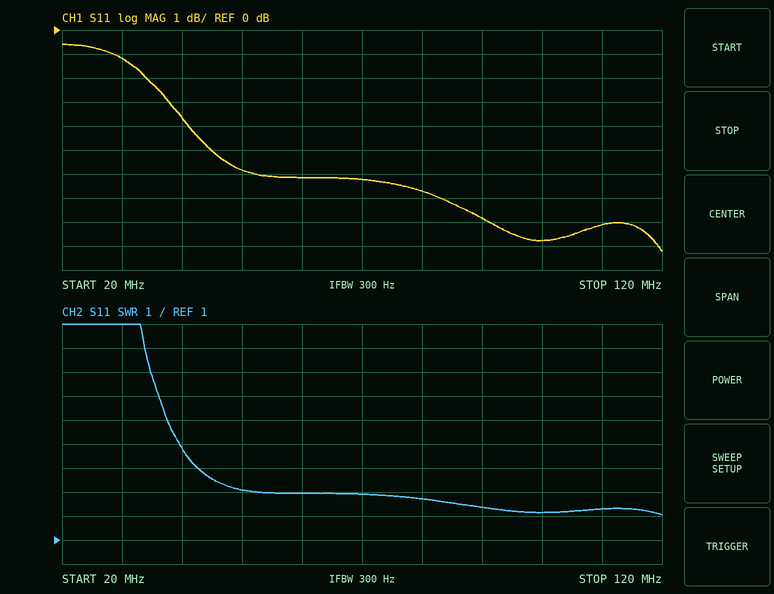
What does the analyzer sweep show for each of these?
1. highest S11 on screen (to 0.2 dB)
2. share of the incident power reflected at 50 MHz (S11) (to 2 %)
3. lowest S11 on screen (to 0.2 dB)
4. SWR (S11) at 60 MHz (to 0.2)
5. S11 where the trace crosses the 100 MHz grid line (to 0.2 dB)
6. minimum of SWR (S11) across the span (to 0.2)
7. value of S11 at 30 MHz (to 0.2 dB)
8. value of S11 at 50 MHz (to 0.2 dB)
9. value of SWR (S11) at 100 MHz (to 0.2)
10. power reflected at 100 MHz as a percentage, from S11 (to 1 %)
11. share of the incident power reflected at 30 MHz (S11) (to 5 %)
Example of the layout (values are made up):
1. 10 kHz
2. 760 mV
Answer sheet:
1. -0.6 dB
2. 26 %
3. -9.2 dB
4. 3.0
5. -8.8 dB
6. 2.0
7. -1.2 dB
8. -5.8 dB
9. 2.2
10. 13 %
11. 75 %
